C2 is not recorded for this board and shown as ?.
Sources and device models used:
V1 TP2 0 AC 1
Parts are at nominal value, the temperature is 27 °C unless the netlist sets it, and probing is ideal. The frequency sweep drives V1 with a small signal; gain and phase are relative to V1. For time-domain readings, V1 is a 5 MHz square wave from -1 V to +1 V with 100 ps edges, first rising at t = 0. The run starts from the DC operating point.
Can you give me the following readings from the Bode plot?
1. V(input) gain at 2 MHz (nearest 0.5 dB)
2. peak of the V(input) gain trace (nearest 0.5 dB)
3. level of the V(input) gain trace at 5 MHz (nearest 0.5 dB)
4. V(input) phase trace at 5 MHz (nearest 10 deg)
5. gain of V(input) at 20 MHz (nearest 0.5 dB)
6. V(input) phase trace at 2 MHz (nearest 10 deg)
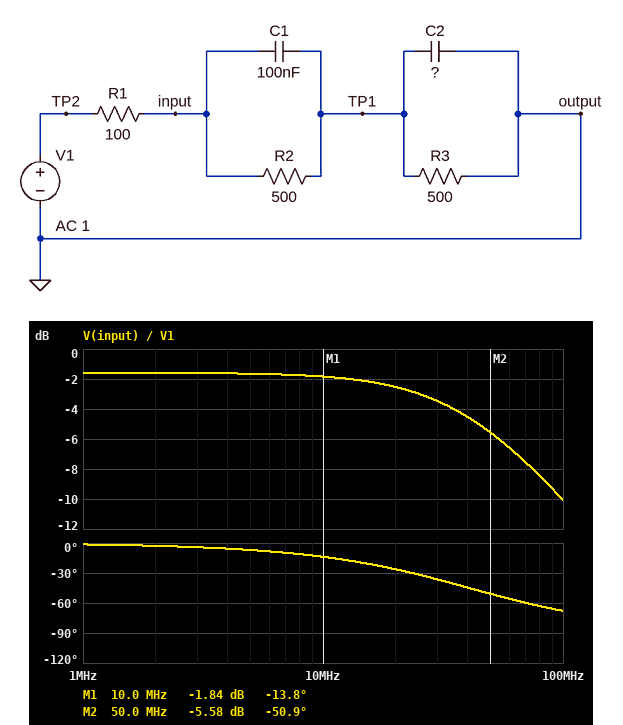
-1.5 dB
-1.5 dB
-1.5 dB
-10 deg
-2.5 dB
0 deg
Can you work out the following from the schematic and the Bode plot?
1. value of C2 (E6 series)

47 pF
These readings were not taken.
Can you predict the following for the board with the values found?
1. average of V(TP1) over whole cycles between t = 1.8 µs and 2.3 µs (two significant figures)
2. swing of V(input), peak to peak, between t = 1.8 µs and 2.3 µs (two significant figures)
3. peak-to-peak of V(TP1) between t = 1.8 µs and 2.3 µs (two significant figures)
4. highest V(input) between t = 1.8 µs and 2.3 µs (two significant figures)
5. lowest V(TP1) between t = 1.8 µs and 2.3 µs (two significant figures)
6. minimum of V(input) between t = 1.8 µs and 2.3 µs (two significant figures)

350 mV
1.7 V
1.7 V
760 mV
-480 mV
-900 mV
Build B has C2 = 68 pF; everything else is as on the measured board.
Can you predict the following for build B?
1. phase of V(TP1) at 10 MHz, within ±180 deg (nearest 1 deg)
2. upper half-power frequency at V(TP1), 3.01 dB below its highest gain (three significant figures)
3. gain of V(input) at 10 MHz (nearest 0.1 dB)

-20 deg
28.1 MHz
-2.1 dB
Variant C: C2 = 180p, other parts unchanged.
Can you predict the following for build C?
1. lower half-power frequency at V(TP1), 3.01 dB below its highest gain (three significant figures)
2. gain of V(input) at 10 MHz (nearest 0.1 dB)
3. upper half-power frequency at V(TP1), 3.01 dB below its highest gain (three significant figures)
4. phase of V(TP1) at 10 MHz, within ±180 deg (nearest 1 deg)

3.70 kHz
-4.3 dB
10.6 MHz
-43 deg
